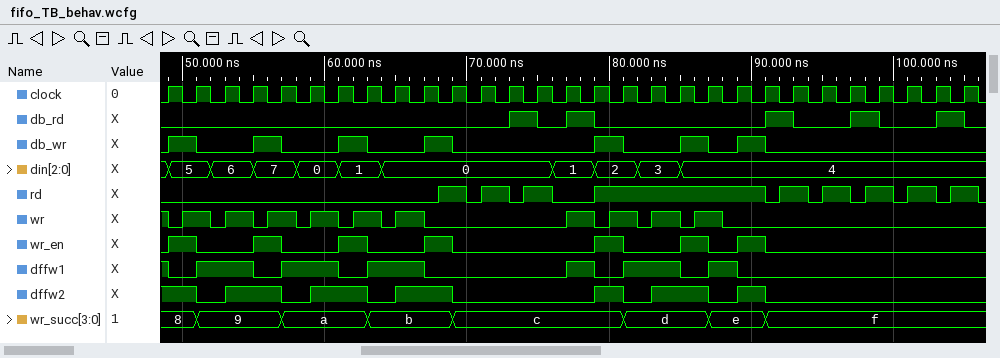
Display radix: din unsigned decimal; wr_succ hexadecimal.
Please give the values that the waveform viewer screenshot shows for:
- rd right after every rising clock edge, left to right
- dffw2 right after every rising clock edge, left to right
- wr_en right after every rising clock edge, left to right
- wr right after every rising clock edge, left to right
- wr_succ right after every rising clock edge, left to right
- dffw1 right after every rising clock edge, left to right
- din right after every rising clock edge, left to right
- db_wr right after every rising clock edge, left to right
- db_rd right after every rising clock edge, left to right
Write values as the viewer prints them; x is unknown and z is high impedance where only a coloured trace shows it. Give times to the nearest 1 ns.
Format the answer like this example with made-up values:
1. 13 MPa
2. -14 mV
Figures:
1. 0 0 0 0 0 0 0 0 0 0 1 1 0 1 0 1 1 1 1 1 1 0 1 1 0 1 1 0 1
2. 1 0 1 1 0 1 1 0 1 1 0 0 0 0 0 1 0 1 1 0 1 0 0 0 0 0 0 0 0
3. 1 0 0 1 0 0 1 0 0 1 0 0 0 0 0 1 0 0 1 0 1 0 0 0 0 0 0 0 0
4. 0 1 1 0 1 1 0 1 1 0 0 0 0 0 1 0 1 1 0 1 0 0 0 0 0 0 0 0 0
5. 8, 9, 9, 9, a, a, a, b, b, b, c, c, c, c, c, c, d, d, d, e, e, f, f, f, f, f, f, f, f
6. 0 1 1 0 1 1 0 1 1 0 0 0 0 0 1 0 1 1 0 1 0 0 0 0 0 0 0 0 0
7. 5, 5, 6, 7, 7, 0, 1, 1, 0, 0, 0, 0, 0, 0, 1, 2, 2, 3, 4, 4, 4, 4, 4, 4, 4, 4, 4, 4, 4
8. 1 0 0 1 0 0 1 0 0 1 0 0 0 0 0 1 0 0 1 0 1 0 0 0 0 0 0 0 0
9. 0 0 0 0 0 0 0 0 0 0 0 0 1 0 1 0 0 0 0 0 0 1 0 0 1 0 0 1 0
